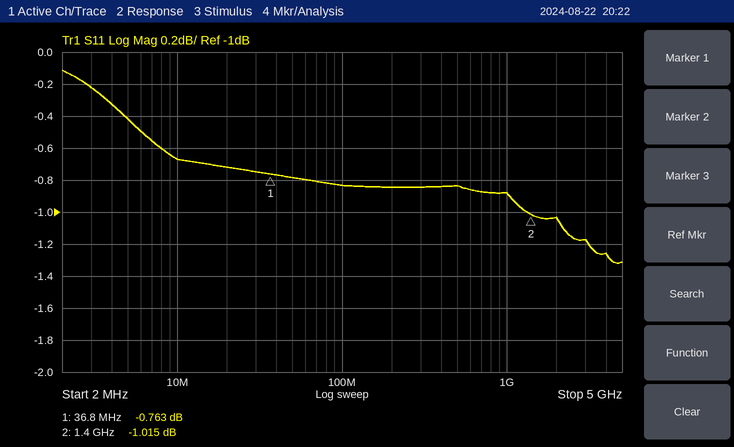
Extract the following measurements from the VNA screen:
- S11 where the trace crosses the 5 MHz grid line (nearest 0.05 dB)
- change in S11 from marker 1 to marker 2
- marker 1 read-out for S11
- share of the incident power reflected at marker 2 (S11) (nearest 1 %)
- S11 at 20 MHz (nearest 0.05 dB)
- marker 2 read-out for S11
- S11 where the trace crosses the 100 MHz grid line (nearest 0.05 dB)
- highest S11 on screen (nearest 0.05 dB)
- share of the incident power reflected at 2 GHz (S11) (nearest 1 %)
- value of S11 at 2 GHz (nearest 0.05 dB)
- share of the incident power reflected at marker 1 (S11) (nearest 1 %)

-0.40 dB
-0.252 dB
-0.763 dB
79 %
-0.70 dB
-1.015 dB
-0.85 dB
-0.10 dB
79 %
-1.05 dB
84 %
